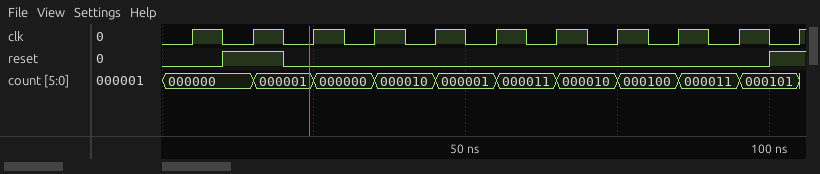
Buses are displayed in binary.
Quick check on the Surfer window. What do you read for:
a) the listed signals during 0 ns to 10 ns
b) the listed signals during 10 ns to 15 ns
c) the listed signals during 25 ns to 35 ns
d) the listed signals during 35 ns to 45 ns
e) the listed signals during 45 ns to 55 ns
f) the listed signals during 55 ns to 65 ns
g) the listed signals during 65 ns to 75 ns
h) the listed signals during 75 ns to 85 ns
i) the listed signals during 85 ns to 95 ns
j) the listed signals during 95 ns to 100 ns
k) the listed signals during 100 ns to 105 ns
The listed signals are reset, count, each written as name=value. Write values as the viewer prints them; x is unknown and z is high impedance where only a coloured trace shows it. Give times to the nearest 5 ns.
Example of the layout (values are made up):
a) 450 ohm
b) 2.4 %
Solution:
a) reset=0, count=000000
b) reset=1, count=000000
c) reset=0, count=000000
d) reset=0, count=000010
e) reset=0, count=000001
f) reset=0, count=000011
g) reset=0, count=000010
h) reset=0, count=000100
i) reset=0, count=000011
j) reset=0, count=000101
k) reset=1, count=000101
